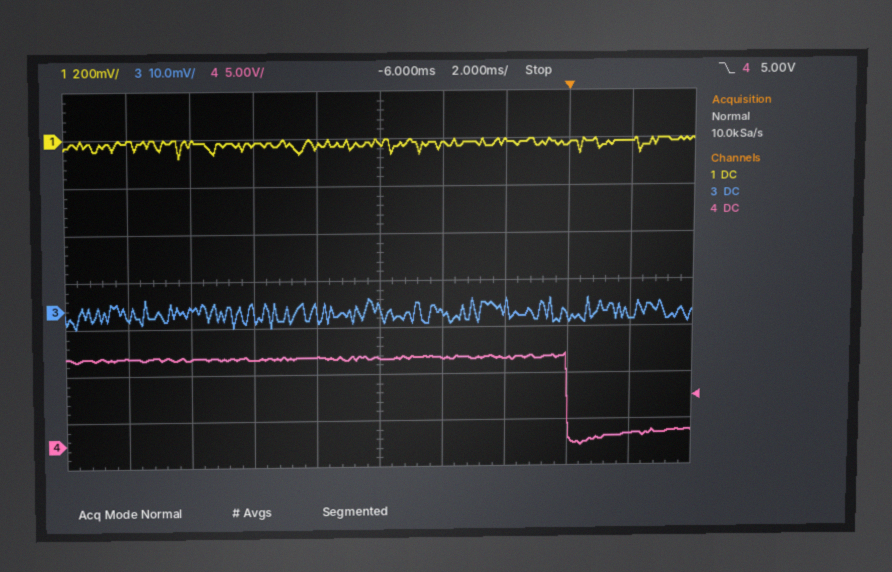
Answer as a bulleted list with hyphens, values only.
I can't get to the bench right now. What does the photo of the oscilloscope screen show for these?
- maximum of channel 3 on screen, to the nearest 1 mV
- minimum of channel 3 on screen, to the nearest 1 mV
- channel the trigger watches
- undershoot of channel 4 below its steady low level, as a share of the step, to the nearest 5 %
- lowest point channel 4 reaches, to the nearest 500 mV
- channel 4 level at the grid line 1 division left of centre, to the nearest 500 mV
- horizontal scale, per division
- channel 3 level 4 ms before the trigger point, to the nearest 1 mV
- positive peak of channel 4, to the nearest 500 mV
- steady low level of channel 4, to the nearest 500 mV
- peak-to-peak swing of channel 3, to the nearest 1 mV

- 2 mV
- -4 mV
- channel 4
- 15 %
- 0.0 V
- 9.5 V
- 2 ms
- -1 mV
- 9.5 V
- 1.0 V
- 6 mV
